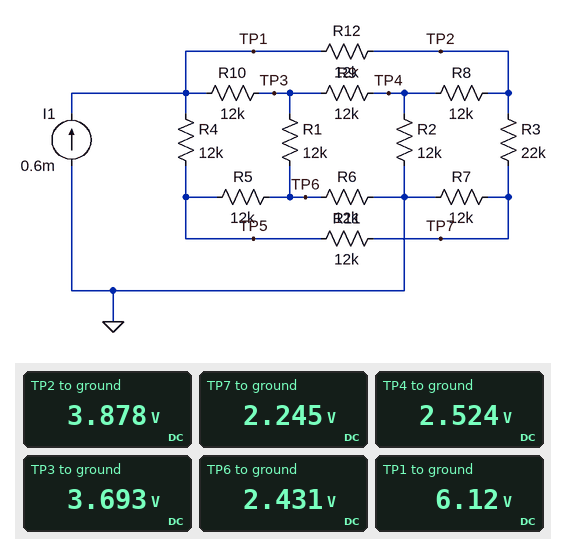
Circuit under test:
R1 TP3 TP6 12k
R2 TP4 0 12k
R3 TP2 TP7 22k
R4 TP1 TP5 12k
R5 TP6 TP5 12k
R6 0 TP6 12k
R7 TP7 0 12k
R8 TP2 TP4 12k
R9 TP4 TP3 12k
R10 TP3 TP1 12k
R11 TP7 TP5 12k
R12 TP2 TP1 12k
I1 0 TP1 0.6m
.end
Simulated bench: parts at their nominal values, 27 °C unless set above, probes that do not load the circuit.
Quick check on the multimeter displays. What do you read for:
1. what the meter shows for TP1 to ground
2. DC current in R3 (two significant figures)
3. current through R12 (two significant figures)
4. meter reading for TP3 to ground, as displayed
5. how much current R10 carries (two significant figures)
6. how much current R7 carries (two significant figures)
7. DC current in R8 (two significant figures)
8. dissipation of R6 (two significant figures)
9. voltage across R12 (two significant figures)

6.12 V
74 µA
190 µA
3.693 V
200 µA
190 µA
110 µA
490 µW
2.2 V
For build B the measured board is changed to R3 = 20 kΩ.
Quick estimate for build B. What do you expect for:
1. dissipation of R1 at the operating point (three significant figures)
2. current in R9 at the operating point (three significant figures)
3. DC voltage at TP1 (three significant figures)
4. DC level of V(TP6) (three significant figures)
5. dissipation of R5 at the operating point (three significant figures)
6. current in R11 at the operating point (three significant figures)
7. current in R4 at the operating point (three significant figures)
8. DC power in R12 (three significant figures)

131 µW
97.8 µA
6.10 V
2.43 V
115 µW
111 µA
209 µA
429 µW
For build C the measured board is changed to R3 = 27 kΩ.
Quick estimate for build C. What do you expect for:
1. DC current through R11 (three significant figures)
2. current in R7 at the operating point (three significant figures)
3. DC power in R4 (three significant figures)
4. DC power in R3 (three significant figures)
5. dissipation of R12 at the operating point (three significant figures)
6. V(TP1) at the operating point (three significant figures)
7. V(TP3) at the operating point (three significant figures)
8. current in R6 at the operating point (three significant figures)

117 µA
183 µA
548 µW
117 µW
401 µW
6.16 V
3.72 V
203 µA
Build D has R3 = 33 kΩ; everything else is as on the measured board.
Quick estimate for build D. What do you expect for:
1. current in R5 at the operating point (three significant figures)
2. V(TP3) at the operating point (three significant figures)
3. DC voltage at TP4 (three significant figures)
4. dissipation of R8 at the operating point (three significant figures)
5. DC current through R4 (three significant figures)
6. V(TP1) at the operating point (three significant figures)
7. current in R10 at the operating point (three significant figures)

95.8 µA
3.75 V
2.60 V
176 µW
217 µA
6.20 V
204 µA
